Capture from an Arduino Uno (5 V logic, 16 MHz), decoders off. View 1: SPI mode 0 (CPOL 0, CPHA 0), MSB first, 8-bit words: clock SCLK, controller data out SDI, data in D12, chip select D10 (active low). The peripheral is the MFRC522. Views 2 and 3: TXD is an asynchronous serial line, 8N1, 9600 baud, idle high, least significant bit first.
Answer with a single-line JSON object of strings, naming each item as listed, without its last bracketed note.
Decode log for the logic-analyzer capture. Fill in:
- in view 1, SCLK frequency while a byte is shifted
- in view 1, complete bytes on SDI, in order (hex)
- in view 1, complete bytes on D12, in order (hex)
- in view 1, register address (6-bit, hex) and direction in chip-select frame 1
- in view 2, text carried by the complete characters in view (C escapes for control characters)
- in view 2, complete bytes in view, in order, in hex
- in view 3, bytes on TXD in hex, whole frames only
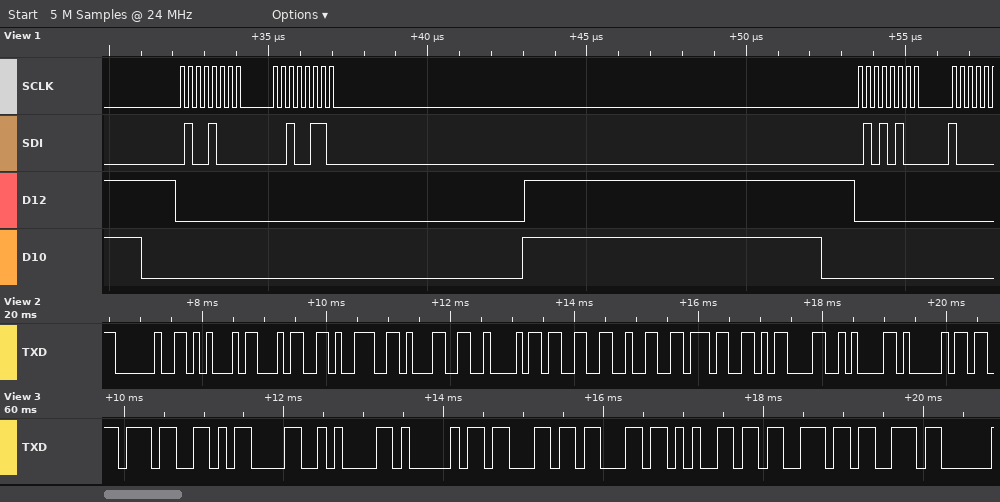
{"in view 1, SCLK frequency while a byte is shifted": "4 MHz", "in view 1, complete bytes on SDI, in order": "48 26 54", "in view 1, complete bytes on D12, in order": "00 00 00", "in view 1, register address (6-bit, hex) and direction in chip-select frame 1": "0x24 write", "in view 2, text carried by the complete characters in view": "\" E491B327\\r\\nA\"", "in view 2, complete bytes in view, in order, in hex": "20 45 34 39 31 42 33 32 37 0D 0A 41", "in view 3, bytes on TXD in hex, whole frames only": "37 0D 0A 41 63 63 65 73 73"}
